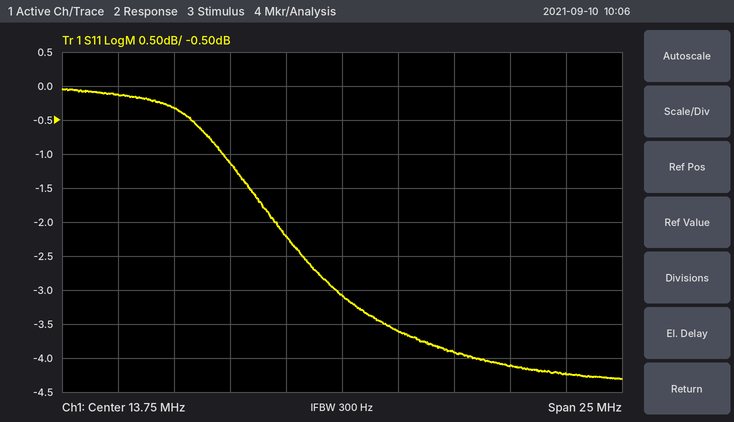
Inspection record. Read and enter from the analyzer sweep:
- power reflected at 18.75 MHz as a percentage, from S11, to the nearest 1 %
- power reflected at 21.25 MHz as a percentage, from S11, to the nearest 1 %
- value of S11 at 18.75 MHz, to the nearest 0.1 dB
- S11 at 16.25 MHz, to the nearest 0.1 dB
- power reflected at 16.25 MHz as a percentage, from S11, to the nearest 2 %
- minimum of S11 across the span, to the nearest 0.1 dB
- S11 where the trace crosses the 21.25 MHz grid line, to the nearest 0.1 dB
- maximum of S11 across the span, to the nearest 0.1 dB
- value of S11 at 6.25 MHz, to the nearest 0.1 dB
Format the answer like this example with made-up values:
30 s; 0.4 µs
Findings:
41 %; 39 %; -3.9 dB; -3.6 dB; 44 %; -4.3 dB; -4.1 dB; 0.0 dB; -0.3 dB
